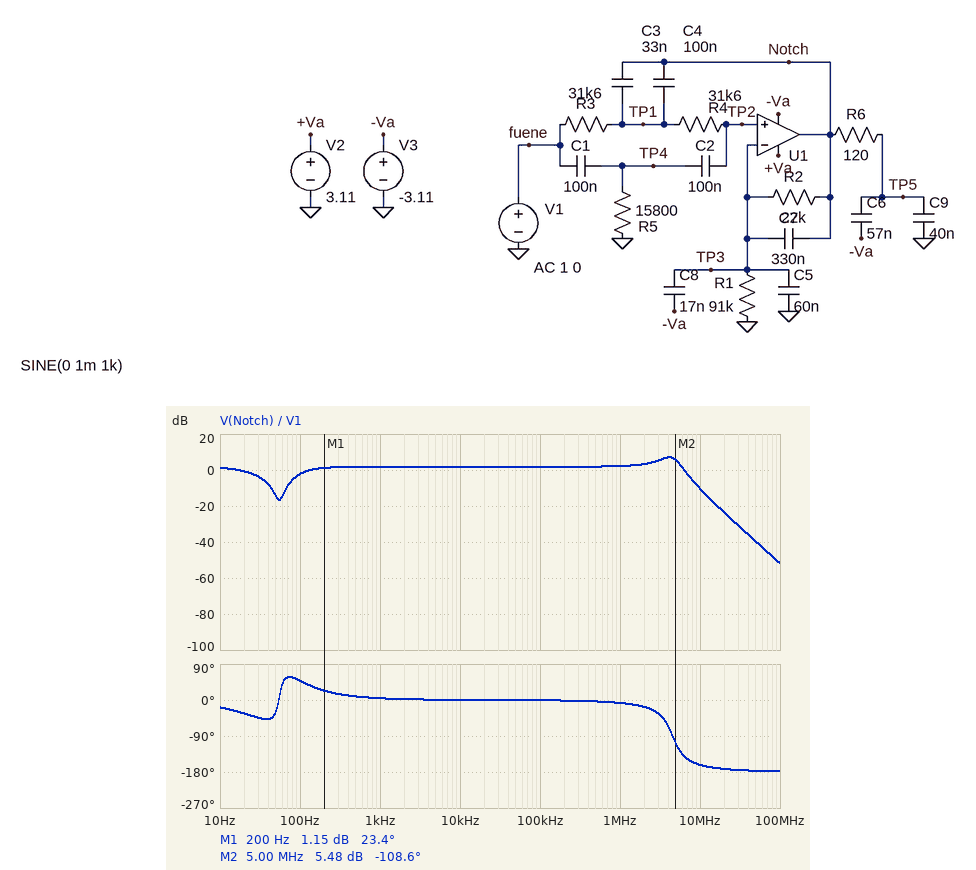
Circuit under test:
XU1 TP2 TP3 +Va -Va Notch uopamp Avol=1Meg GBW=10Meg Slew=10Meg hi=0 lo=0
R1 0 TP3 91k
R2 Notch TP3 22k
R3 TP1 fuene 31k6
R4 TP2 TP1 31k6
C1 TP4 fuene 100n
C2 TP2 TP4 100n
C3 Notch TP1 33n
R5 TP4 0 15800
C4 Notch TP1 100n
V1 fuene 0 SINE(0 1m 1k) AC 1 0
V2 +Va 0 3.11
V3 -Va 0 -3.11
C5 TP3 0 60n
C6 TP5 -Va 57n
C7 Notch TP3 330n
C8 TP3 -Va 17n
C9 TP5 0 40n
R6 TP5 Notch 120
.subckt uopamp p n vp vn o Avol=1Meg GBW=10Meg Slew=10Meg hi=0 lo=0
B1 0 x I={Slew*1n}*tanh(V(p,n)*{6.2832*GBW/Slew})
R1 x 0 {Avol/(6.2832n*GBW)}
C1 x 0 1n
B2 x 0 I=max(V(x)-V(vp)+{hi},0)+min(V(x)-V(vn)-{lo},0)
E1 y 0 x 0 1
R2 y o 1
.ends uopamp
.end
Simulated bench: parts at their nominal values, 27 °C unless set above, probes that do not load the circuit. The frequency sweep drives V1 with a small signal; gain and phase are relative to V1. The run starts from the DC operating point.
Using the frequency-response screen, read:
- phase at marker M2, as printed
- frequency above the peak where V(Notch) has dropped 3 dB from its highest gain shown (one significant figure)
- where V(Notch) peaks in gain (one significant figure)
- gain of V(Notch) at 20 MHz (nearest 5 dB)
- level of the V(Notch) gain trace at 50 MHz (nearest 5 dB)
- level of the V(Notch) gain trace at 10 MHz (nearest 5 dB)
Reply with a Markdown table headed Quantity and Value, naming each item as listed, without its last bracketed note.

| Quantity | Value |
|---|---|
| phase at marker M2, as printed | -108.6 deg |
| frequency above the peak where V(Notch) has dropped 3 dB from its highest gain shown | 5 MHz |
| where V(Notch) peaks in gain | 4 MHz |
| gain of V(Notch) at 20 MHz | -25 dB |
| level of the V(Notch) gain trace at 50 MHz | -40 dB |
| level of the V(Notch) gain trace at 10 MHz | -10 dB |
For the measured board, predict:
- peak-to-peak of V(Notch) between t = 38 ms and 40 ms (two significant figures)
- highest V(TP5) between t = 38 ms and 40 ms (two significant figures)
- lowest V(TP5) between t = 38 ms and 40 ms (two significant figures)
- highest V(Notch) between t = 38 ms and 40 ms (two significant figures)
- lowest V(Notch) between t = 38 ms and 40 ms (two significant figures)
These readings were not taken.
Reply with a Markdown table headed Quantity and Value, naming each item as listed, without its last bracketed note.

| Quantity | Value |
|---|---|
| peak-to-peak of V(Notch) between t = 38 ms and 40 ms | 2.5 mV |
| highest V(TP5) between t = 38 ms and 40 ms | 1.2 mV |
| lowest V(TP5) between t = 38 ms and 40 ms | -1.2 mV |
| highest V(Notch) between t = 38 ms and 40 ms | 1.2 mV |
| lowest V(Notch) between t = 38 ms and 40 ms | -1.2 mV |
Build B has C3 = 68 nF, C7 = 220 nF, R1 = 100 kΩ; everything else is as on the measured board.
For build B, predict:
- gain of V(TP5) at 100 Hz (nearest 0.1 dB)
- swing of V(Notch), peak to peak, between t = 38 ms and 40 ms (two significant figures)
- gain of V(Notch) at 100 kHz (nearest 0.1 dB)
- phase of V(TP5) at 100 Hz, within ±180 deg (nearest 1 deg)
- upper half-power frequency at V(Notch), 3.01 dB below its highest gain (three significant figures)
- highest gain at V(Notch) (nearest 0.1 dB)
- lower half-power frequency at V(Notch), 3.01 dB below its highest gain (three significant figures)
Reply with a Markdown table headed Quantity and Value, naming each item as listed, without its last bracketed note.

| Quantity | Value |
|---|---|
| gain of V(TP5) at 100 Hz | -0.1 dB |
| swing of V(Notch), peak to peak, between t = 38 ms and 40 ms | 2.7 mV |
| gain of V(Notch) at 100 kHz | 2.6 dB |
| phase of V(TP5) at 100 Hz, within ±180 deg | 47 deg |
| upper half-power frequency at V(Notch), 3.01 dB below its highest gain | 5.37 MHz |
| highest gain at V(Notch) | 7.2 dB |
| lower half-power frequency at V(Notch), 3.01 dB below its highest gain | 2.13 MHz |
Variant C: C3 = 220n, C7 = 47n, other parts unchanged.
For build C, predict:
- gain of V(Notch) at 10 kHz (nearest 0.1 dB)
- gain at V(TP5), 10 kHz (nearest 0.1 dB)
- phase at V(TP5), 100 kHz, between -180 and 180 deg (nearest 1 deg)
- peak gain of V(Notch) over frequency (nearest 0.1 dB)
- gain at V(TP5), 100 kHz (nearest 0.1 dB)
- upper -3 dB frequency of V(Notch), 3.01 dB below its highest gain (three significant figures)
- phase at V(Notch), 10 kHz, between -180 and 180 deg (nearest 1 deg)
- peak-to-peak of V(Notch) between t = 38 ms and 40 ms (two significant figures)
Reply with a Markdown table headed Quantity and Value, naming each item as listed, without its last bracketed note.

| Quantity | Value |
|---|---|
| gain of V(Notch) at 10 kHz | 8.4 dB |
| gain at V(TP5), 10 kHz | 6.6 dB |
| phase at V(TP5), 100 kHz, between -180 and 180 deg | -84 deg |
| peak gain of V(Notch) over frequency | 13.3 dB |
| gain at V(TP5), 100 kHz | -8.9 dB |
| upper -3 dB frequency of V(Notch), 3.01 dB below its highest gain | 184 Hz |
| phase at V(Notch), 10 kHz, between -180 and 180 deg | 0 deg |
| peak-to-peak of V(Notch) between t = 38 ms and 40 ms | 5.3 mV |
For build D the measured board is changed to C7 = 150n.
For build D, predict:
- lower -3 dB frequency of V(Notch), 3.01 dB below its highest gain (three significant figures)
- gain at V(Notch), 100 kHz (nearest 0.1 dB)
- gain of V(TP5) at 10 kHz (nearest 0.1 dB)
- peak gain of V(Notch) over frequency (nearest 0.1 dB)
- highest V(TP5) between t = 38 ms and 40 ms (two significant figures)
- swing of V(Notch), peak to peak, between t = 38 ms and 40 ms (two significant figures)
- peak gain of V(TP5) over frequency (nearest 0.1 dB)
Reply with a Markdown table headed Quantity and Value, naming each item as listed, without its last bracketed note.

| Quantity | Value |
|---|---|
| lower -3 dB frequency of V(Notch), 3.01 dB below its highest gain | 1.50 MHz |
| gain at V(Notch), 100 kHz | 3.6 dB |
| gain of V(TP5) at 10 kHz | 1.7 dB |
| peak gain of V(Notch) over frequency | 7.3 dB |
| highest V(TP5) between t = 38 ms and 40 ms | 1.5 mV |
| swing of V(Notch), peak to peak, between t = 38 ms and 40 ms | 3.0 mV |
| peak gain of V(TP5) over frequency | 3.7 dB |
